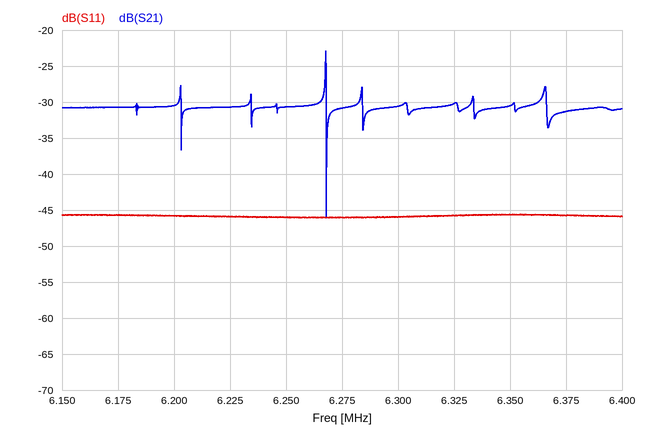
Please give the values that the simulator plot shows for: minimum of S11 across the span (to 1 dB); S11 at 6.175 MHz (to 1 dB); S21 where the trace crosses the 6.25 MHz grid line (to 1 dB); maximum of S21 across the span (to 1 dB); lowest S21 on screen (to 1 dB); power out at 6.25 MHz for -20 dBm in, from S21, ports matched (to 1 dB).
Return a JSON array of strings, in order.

["-46 dB", "-46 dB", "-31 dB", "-23 dB", "-46 dB", "-51 dBm"]
